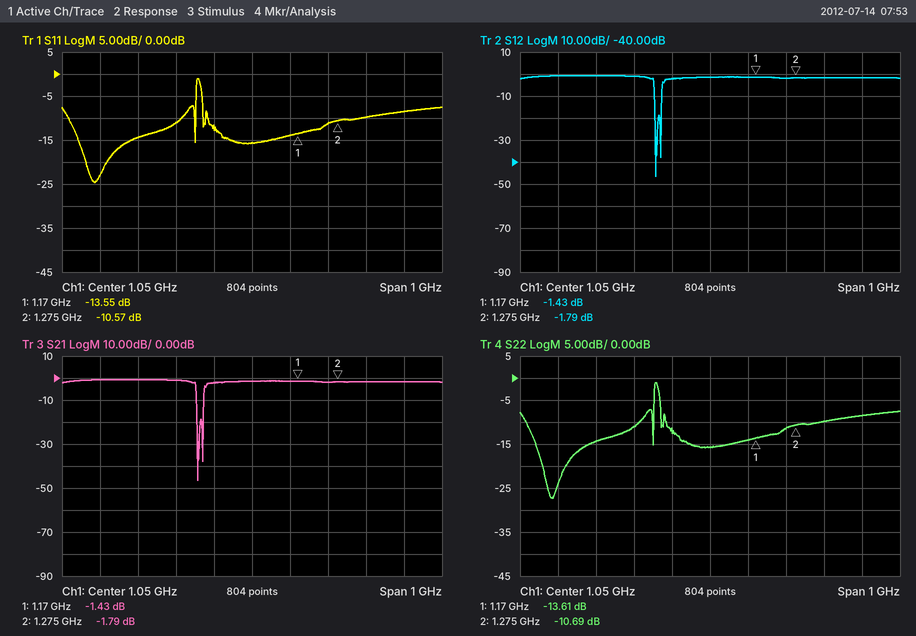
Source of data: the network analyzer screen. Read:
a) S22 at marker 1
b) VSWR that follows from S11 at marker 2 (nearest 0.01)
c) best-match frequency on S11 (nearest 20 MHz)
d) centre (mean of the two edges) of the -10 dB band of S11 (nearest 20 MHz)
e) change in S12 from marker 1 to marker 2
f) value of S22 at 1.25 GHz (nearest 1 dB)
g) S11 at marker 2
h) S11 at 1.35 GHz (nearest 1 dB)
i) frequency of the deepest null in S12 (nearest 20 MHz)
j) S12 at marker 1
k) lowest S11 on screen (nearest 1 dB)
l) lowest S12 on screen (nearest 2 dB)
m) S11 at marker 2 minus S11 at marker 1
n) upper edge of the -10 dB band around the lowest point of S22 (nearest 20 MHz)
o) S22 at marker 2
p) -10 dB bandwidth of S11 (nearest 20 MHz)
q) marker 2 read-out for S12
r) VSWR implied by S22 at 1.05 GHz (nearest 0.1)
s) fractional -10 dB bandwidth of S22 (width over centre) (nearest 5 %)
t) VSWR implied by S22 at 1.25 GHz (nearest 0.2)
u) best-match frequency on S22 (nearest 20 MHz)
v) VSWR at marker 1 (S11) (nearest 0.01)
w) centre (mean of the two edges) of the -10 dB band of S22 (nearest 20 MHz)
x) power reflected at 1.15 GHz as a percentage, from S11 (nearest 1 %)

-13.61 dB
1.84
640 MHz
720 MHz
-0.36 dB
-11 dB
-10.57 dB
-10 dB
900 MHz
-1.43 dB
-25 dB
-46 dB
2.98 dB
860 MHz
-10.69 dB
300 MHz
-1.79 dB
1.4
40 %
1.8
640 MHz
1.53
720 MHz
4 %
